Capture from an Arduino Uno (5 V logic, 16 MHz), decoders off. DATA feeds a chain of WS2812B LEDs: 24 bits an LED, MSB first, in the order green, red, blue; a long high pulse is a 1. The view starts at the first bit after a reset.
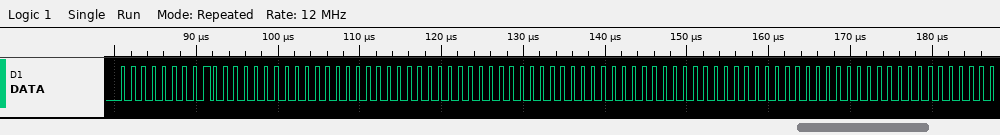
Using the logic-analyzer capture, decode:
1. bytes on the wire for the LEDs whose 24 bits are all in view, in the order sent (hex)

00 80 00 00 00 00 00 00 00
